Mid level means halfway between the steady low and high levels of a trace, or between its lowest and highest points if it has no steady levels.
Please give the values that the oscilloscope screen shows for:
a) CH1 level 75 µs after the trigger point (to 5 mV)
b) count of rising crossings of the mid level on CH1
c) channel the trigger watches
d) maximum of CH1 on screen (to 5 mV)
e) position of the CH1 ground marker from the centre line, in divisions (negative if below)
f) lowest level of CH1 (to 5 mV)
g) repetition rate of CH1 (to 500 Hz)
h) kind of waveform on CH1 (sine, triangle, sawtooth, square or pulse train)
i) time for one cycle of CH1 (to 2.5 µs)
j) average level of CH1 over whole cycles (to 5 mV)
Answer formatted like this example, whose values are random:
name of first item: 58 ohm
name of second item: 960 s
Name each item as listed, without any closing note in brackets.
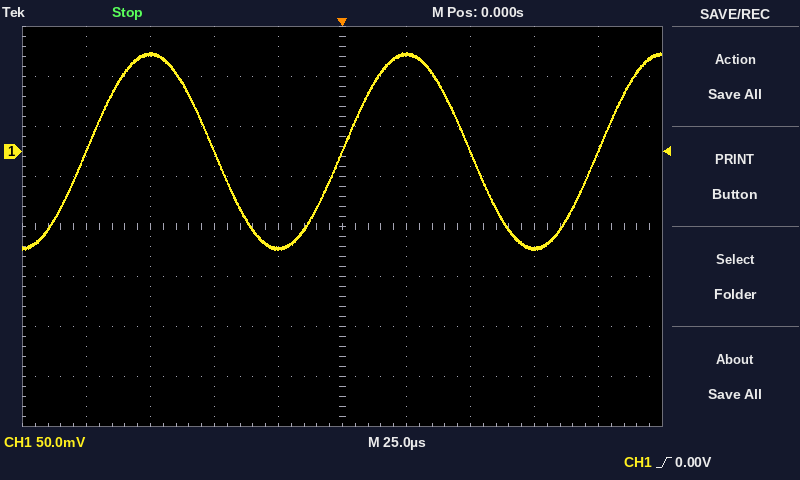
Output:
CH1 level 75 µs after the trigger point: -95 mV
count of rising crossings of the mid level on CH1: 3
channel the trigger watches: CH1
maximum of CH1 on screen: 100 mV
position of the CH1 ground marker from the centre line, in divisions: +1.5 div
lowest level of CH1: -100 mV
repetition rate of CH1: 10.0 kHz
kind of waveform on CH1: sine
time for one cycle of CH1: 100.0 µs
average level of CH1 over whole cycles: 0 mV
